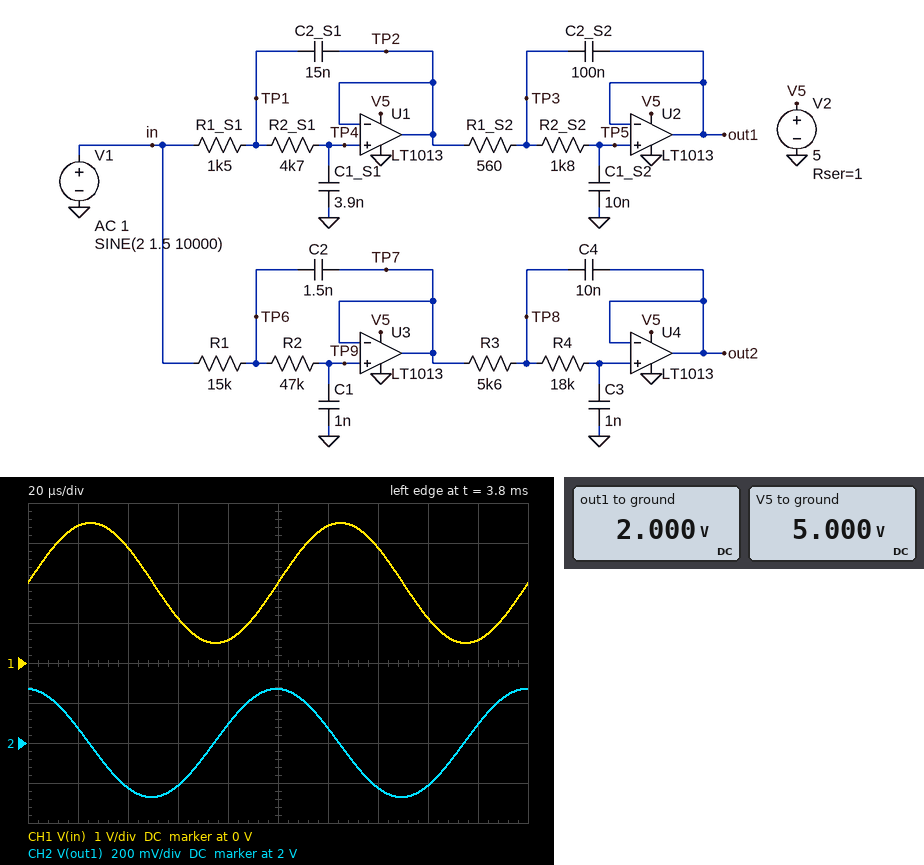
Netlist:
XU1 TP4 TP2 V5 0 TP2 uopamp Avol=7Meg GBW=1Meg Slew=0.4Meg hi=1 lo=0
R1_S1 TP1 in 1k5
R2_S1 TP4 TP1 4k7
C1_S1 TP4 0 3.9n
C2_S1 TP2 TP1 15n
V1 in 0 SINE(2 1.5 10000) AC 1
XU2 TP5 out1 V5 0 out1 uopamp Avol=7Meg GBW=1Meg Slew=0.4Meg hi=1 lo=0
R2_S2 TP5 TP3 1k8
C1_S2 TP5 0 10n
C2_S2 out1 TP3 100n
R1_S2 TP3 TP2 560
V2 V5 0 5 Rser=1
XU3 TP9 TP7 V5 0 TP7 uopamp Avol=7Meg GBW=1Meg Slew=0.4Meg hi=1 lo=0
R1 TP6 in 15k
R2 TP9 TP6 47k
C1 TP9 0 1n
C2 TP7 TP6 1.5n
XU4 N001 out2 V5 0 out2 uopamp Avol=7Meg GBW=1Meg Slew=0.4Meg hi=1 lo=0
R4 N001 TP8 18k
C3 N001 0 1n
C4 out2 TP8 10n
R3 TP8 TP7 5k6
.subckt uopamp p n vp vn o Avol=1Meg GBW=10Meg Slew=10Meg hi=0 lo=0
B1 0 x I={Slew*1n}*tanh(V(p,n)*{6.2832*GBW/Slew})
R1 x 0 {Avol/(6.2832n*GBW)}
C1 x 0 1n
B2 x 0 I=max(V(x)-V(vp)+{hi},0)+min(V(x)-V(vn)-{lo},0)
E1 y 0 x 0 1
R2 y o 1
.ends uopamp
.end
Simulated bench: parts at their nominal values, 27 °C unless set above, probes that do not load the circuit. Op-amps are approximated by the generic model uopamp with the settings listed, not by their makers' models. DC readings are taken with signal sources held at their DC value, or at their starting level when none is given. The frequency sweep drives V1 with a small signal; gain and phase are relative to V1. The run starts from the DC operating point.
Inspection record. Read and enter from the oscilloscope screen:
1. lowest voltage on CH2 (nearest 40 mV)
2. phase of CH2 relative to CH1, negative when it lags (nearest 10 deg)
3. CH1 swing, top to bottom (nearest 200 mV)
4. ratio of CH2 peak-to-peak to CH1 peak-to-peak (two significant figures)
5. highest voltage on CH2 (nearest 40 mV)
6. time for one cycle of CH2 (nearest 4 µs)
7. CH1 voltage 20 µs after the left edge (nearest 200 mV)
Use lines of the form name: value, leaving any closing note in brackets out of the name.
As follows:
lowest voltage on CH2: 1.72 V
phase of CH2 relative to CH1, negative when it lags: 90 deg
CH1 swing, top to bottom: 3.0 V
ratio of CH2 peak-to-peak to CH1 peak-to-peak: 0.18
highest voltage on CH2: 2.28 V
time for one cycle of CH2: 100 µs
CH1 voltage 20 µs after the left edge: 3.4 V
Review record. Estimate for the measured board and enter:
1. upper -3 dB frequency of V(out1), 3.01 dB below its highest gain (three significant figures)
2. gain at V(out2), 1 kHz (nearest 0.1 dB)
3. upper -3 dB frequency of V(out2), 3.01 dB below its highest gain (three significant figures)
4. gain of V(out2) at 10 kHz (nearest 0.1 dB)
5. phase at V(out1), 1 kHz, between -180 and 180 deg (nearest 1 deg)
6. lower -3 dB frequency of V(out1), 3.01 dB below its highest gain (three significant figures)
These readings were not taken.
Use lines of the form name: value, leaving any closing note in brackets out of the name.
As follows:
upper -3 dB frequency of V(out1), 3.01 dB below its highest gain: 5.83 kHz
gain at V(out2), 1 kHz: 0 dB
upper -3 dB frequency of V(out2), 3.01 dB below its highest gain: 4.95 kHz
gain of V(out2) at 10 kHz: -24.6 dB
phase at V(out1), 1 kHz, between -180 and 180 deg: -18 deg
lower -3 dB frequency of V(out1), 3.01 dB below its highest gain: 1.48 kHz
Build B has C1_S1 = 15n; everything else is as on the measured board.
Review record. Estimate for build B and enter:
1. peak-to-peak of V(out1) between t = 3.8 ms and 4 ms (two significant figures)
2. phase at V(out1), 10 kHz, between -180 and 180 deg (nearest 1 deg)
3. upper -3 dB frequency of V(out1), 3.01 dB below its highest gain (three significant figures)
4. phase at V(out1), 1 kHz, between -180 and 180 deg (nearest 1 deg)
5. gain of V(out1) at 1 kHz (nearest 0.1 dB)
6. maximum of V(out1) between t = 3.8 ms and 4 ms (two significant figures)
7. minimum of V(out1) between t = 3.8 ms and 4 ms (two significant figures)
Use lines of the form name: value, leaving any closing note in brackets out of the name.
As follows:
peak-to-peak of V(out1) between t = 3.8 ms and 4 ms: 110 mV
phase at V(out1), 10 kHz, between -180 and 180 deg: 73 deg
upper -3 dB frequency of V(out1), 3.01 dB below its highest gain: 3.05 kHz
phase at V(out1), 1 kHz, between -180 and 180 deg: -41 deg
gain of V(out1) at 1 kHz: -0.6 dB
maximum of V(out1) between t = 3.8 ms and 4 ms: 2.1 V
minimum of V(out1) between t = 3.8 ms and 4 ms: 1.9 V
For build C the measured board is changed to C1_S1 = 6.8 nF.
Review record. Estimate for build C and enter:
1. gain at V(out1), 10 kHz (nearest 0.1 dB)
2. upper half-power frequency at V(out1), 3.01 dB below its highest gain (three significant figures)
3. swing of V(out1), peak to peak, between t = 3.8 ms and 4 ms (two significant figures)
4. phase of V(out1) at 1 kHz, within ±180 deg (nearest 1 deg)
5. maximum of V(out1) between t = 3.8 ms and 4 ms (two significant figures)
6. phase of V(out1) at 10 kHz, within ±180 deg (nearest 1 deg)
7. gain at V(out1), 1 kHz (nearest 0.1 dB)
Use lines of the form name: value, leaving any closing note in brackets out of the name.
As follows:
gain at V(out1), 10 kHz: -20.7 dB
upper half-power frequency at V(out1), 3.01 dB below its highest gain: 5.36 kHz
swing of V(out1), peak to peak, between t = 3.8 ms and 4 ms: 280 mV
phase of V(out1) at 1 kHz, within ±180 deg: -24 deg
maximum of V(out1) between t = 3.8 ms and 4 ms: 2.1 V
phase of V(out1) at 10 kHz, within ±180 deg: 80 deg
gain at V(out1), 1 kHz: 0.2 dB
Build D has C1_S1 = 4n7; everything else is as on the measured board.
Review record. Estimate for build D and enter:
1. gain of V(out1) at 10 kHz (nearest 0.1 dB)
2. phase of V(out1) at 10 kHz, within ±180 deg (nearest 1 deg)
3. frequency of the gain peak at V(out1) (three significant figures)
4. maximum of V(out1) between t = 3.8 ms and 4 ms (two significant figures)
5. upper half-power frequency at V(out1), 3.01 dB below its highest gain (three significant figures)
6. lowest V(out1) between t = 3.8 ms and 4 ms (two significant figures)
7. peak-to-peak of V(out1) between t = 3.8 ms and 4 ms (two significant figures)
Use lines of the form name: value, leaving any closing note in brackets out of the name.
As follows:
gain of V(out1) at 10 kHz: -16.9 dB
phase of V(out1) at 10 kHz, within ±180 deg: 87 deg
frequency of the gain peak at V(out1): 4.13 kHz
maximum of V(out1) between t = 3.8 ms and 4 ms: 2.2 V
upper half-power frequency at V(out1), 3.01 dB below its highest gain: 5.67 kHz
lowest V(out1) between t = 3.8 ms and 4 ms: 1.8 V
peak-to-peak of V(out1) between t = 3.8 ms and 4 ms: 430 mV
